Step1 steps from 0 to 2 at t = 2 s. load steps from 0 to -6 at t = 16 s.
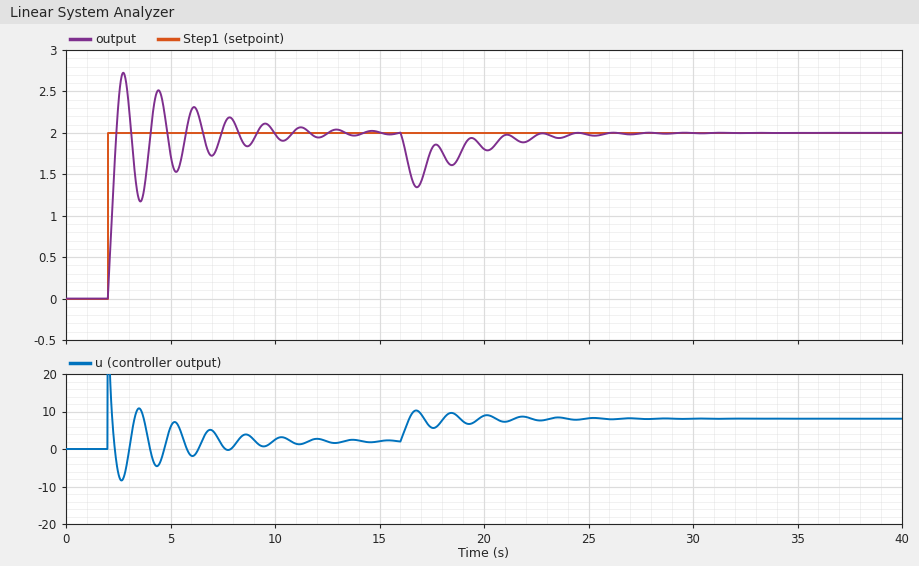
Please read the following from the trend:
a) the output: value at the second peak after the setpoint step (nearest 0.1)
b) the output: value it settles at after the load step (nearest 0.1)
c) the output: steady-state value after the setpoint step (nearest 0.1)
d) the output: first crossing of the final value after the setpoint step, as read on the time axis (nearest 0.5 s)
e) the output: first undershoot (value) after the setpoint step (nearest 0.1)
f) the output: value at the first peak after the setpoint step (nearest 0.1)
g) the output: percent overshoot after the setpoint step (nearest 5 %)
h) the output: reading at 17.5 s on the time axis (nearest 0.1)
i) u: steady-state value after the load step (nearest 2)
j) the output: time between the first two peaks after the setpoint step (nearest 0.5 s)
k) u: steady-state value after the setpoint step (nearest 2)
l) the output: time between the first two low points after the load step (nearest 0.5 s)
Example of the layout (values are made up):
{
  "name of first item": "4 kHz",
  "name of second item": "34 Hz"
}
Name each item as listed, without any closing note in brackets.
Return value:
{
  "the output: value at the second peak after the setpoint step": "2.5",
  "the output: value it settles at after the load step": "2.0",
  "the output: steady-state value after the setpoint step": "2.0",
  "the output: first crossing of the final value after the setpoint step, as read on the time axis": "2.5 s",
  "the output: first undershoot (value) after the setpoint step": "1.2",
  "the output: value at the first peak after the setpoint step": "2.7",
  "the output: percent overshoot after the setpoint step": "35 %",
  "the output: reading at 17.5 s on the time axis": "1.8",
  "u: steady-state value after the load step": "8",
  "the output: time between the first two peaks after the setpoint step": "1.5 s",
  "u: steady-state value after the setpoint step": "2",
  "the output: time between the first two low points after the load step": "1.5 s"
}
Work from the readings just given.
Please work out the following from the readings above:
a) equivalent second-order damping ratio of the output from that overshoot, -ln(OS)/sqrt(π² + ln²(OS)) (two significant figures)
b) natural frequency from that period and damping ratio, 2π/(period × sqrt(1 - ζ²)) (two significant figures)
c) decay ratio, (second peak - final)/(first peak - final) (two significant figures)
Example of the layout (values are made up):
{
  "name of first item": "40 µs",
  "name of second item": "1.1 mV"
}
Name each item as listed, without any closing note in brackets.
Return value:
{
  "equivalent second-order damping ratio of the output from that overshoot, -ln(OS)/sqrt(π² + ln²(OS))": "0.32",
  "natural frequency from that period and damping ratio, 2π/(period × sqrt(1 - ζ²))": "4.4 rad/s",
  "decay ratio, (second peak - final)/(first peak - final)": "0.71"
}
